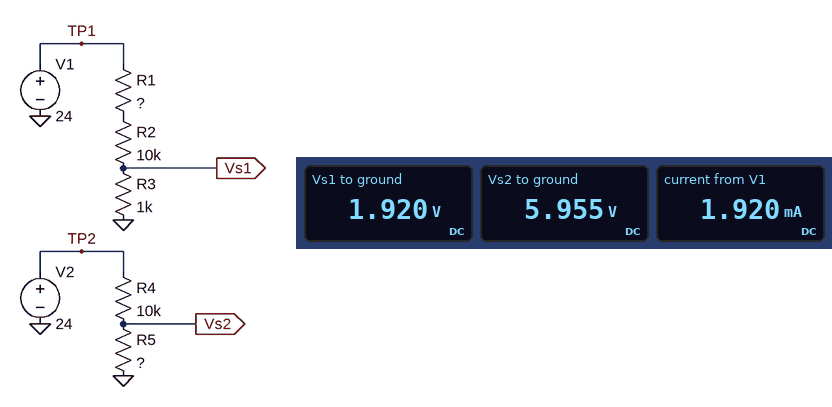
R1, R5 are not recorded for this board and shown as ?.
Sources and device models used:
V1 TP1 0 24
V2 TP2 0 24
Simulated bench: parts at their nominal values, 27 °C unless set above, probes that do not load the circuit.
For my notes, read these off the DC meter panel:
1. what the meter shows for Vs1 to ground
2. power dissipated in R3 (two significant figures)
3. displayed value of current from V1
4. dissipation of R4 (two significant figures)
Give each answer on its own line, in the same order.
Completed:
1.920 V
3.7 mW
1.920 mA
33 mW
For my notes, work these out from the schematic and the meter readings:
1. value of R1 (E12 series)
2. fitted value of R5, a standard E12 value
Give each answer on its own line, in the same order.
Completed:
1.5 kΩ
3.3 kΩ
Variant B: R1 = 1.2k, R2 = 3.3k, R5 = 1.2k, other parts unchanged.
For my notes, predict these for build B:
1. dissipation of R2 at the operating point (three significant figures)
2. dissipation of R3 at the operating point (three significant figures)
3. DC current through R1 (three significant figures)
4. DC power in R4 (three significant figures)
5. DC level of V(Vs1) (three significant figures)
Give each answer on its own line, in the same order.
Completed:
62.8 mW
19.0 mW
4.36 mA
45.9 mW
4.36 V
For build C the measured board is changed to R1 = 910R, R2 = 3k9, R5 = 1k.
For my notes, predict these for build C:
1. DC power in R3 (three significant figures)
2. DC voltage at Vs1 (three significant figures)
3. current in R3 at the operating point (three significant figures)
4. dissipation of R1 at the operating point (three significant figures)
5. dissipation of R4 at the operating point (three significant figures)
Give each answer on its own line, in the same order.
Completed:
17.1 mW
4.13 V
4.13 mA
15.5 mW
47.6 mW
